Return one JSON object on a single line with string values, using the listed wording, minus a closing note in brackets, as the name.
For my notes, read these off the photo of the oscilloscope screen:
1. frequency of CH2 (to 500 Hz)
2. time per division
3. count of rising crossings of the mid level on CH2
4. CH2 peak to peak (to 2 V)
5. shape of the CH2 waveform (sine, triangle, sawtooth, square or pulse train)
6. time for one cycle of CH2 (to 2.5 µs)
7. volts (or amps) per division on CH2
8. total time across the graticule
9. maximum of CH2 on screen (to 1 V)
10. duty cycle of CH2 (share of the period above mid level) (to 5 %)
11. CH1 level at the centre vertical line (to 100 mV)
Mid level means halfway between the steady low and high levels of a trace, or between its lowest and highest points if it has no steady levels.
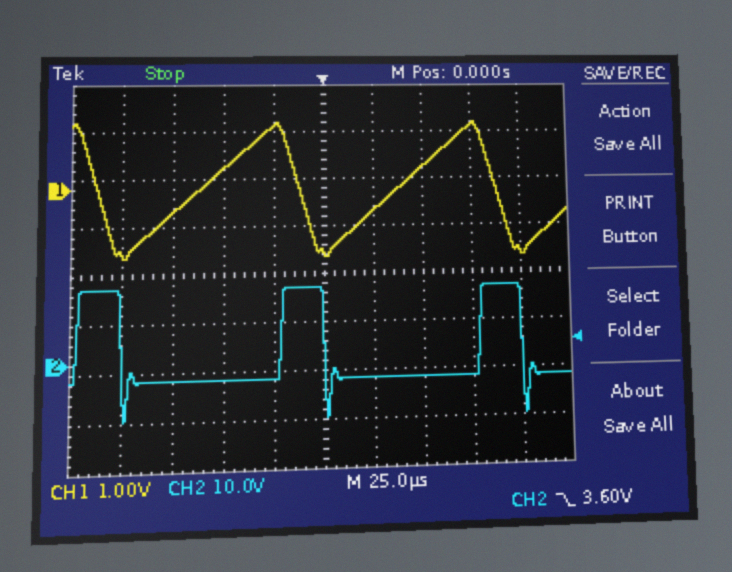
{"frequency of CH2": "10.0 kHz", "time per division": "25 µs", "count of rising crossings of the mid level on CH2": "3", "CH2 peak to peak": "26 V", "shape of the CH2 waveform": "pulse train", "time for one cycle of CH2": "100.0 µs", "volts (or amps) per division on CH2": "10 V", "total time across the graticule": "250 µs", "maximum of CH2 on screen": "15 V", "duty cycle of CH2 (share of the period above mid level)": "20 %", "CH1 level at the centre vertical line": "-1.4 V"}
